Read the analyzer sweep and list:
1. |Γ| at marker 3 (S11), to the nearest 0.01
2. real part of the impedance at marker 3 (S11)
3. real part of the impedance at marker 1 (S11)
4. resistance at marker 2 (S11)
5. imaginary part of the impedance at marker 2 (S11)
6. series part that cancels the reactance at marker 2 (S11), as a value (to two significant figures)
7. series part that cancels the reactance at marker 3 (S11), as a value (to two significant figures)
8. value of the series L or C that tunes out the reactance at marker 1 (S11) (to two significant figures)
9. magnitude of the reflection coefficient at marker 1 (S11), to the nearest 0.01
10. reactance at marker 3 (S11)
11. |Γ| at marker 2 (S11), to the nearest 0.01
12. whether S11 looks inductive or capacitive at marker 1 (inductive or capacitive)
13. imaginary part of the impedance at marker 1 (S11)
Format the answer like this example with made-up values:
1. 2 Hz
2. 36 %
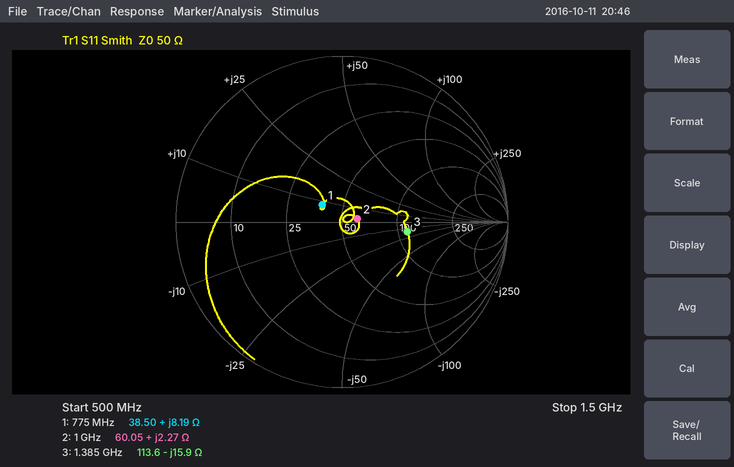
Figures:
1. 0.40
2. 113.6 Ω
3. 38.50 Ω
4. 60.05 Ω
5. +2.27 Ω
6. 70 pF
7. 1.8 nH
8. 25 pF
9. 0.16
10. -15.9 Ω
11. 0.09
12. inductive
13. +8.19 Ω
